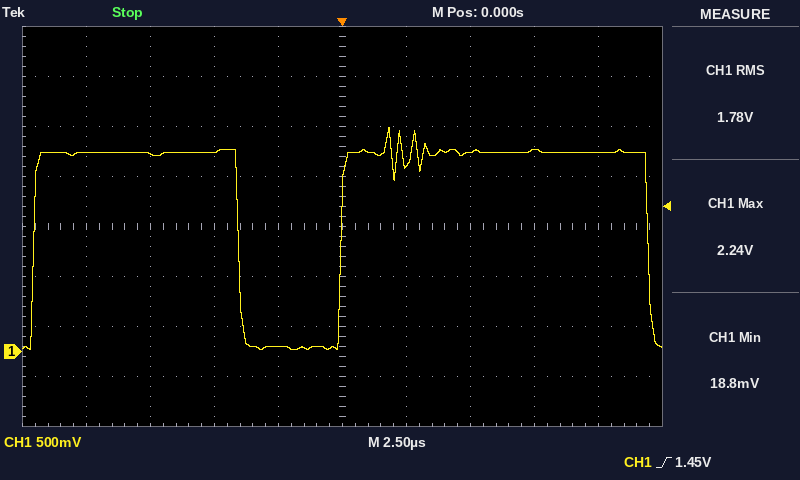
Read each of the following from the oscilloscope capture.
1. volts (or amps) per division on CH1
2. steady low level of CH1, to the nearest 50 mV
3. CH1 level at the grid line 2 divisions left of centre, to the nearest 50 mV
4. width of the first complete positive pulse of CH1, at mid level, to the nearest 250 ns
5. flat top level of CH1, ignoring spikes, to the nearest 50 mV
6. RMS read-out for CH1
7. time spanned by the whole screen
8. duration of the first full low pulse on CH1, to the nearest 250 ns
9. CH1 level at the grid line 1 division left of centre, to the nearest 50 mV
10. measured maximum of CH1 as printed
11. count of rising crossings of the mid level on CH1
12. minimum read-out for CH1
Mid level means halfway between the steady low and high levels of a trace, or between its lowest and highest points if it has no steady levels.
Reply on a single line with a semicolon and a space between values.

500 mV; 50 mV; 2.00 V; 8.00 µs; 2.00 V; 1.78 V; 25 µs; 4.00 µs; 50 mV; 2.24 V; 2; 18.8 mV
